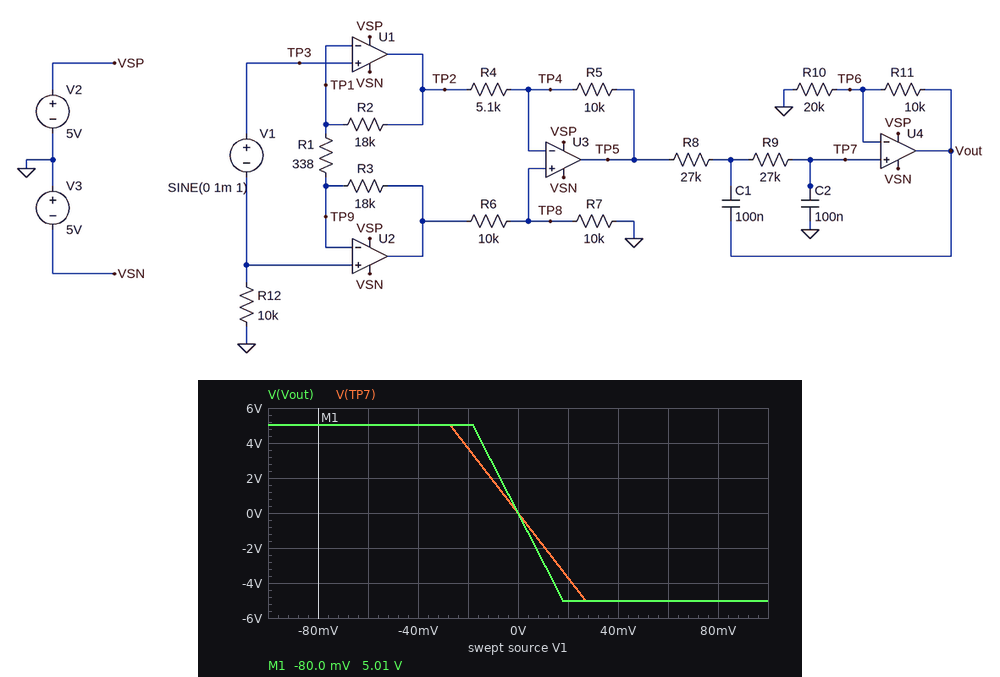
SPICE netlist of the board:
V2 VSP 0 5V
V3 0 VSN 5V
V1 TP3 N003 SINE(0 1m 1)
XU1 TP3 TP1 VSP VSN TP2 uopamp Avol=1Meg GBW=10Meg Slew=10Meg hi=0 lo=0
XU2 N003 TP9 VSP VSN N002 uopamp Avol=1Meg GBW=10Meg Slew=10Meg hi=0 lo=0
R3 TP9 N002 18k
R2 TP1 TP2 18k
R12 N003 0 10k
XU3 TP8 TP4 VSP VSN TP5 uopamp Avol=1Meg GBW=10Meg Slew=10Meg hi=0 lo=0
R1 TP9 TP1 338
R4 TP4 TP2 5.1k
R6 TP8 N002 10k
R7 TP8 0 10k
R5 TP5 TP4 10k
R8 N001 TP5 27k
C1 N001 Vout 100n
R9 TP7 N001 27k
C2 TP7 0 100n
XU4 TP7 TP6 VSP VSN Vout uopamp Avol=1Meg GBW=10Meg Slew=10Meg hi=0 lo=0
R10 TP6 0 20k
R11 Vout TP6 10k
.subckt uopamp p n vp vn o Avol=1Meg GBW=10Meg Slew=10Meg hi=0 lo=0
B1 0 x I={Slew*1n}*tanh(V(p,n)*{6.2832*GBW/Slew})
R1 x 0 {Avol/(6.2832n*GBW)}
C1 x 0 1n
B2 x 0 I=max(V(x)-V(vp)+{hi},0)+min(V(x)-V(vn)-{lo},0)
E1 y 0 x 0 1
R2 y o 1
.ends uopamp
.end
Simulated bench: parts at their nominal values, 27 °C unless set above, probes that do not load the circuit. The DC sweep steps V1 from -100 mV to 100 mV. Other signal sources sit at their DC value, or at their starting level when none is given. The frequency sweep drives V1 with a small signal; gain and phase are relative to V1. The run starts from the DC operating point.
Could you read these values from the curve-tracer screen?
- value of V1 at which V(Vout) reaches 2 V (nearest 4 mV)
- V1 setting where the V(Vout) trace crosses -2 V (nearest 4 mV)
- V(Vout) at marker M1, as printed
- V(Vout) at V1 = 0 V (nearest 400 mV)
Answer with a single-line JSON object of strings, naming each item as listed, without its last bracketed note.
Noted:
{"value of V1 at which V(Vout) reaches 2 V": "-8 mV", "V1 setting where the V(Vout) trace crosses -2 V": "8 mV", "V(Vout) at marker M1, as printed": "5.01 V", "V(Vout) at V1 = 0 V": "0 V"}
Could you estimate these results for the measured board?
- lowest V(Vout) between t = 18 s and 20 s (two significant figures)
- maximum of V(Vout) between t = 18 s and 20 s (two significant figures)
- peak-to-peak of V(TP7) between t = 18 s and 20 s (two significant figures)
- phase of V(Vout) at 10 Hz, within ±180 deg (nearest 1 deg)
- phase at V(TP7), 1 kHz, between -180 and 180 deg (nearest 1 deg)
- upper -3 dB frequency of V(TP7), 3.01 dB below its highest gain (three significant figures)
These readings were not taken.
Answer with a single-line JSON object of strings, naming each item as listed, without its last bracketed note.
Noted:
{"lowest V(Vout) between t = 18 s and 20 s": "-280 mV", "maximum of V(Vout) between t = 18 s and 20 s": "280 mV", "peak-to-peak of V(TP7) between t = 18 s and 20 s": "370 mV", "phase of V(Vout) at 10 Hz, within ±180 deg": "165 deg", "phase at V(TP7), 1 kHz, between -180 and 180 deg": "4 deg", "upper -3 dB frequency of V(TP7), 3.01 dB below its highest gain": "55.4 Hz"}
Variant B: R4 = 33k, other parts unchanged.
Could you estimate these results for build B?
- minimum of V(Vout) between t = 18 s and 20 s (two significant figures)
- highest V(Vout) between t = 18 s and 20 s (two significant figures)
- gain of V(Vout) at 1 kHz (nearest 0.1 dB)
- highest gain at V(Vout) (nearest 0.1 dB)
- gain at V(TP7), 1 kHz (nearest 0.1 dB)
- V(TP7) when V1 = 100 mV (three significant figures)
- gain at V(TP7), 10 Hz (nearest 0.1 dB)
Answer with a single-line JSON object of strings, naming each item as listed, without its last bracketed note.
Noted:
{"minimum of V(Vout) between t = 18 s and 20 s": "-77 mV", "highest V(Vout) between t = 18 s and 20 s": "77 mV", "gain of V(Vout) at 1 kHz": "-11.5 dB", "highest gain at V(Vout)": "37.7 dB", "gain at V(TP7), 1 kHz": "-15.0 dB", "V(TP7) when V1 = 100 mV": "-4.71 V", "gain at V(TP7), 10 Hz": "34.1 dB"}
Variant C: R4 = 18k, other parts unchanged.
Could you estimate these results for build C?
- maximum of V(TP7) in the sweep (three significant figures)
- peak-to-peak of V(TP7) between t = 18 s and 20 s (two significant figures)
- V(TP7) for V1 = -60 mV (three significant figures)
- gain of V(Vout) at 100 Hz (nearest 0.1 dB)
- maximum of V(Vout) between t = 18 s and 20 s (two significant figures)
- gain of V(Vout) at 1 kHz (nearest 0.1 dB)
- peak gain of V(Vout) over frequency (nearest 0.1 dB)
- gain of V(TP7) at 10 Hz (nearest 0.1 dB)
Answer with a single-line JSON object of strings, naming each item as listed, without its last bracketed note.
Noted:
{"maximum of V(TP7) in the sweep": "5.01 V", "peak-to-peak of V(TP7) between t = 18 s and 20 s": "140 mV", "V(TP7) for V1 = -60 mV": "4.29 V", "gain of V(Vout) at 100 Hz": "30.6 dB", "maximum of V(Vout) between t = 18 s and 20 s": "110 mV", "gain of V(Vout) at 1 kHz": "-8.6 dB", "peak gain of V(Vout) over frequency": "40.6 dB", "gain of V(TP7) at 10 Hz": "37.1 dB"}
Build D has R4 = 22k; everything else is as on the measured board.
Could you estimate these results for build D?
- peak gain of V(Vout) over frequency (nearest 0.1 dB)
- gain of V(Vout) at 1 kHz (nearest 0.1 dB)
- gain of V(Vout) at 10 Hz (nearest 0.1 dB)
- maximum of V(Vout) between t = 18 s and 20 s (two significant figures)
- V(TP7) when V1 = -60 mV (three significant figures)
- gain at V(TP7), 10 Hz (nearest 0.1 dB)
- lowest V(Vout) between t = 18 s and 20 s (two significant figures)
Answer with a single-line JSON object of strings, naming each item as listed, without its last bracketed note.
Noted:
{"peak gain of V(Vout) over frequency": "39.6 dB", "gain of V(Vout) at 1 kHz": "-9.6 dB", "gain of V(Vout) at 10 Hz": "39.5 dB", "maximum of V(Vout) between t = 18 s and 20 s": "95 mV", "V(TP7) when V1 = -60 mV": "3.80 V", "gain at V(TP7), 10 Hz": "36.0 dB", "lowest V(Vout) between t = 18 s and 20 s": "-95 mV"}
